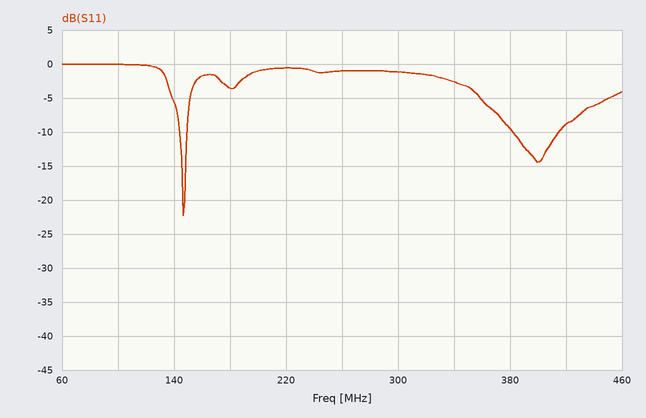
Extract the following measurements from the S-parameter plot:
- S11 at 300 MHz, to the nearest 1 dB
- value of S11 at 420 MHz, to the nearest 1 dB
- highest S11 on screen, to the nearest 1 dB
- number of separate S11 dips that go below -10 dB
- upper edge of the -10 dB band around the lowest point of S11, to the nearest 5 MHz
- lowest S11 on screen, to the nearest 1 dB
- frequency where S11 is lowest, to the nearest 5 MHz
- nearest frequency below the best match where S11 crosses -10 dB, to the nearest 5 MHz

-1 dB
-9 dB
0 dB
2
150 MHz
-22 dB
145 MHz
145 MHz
